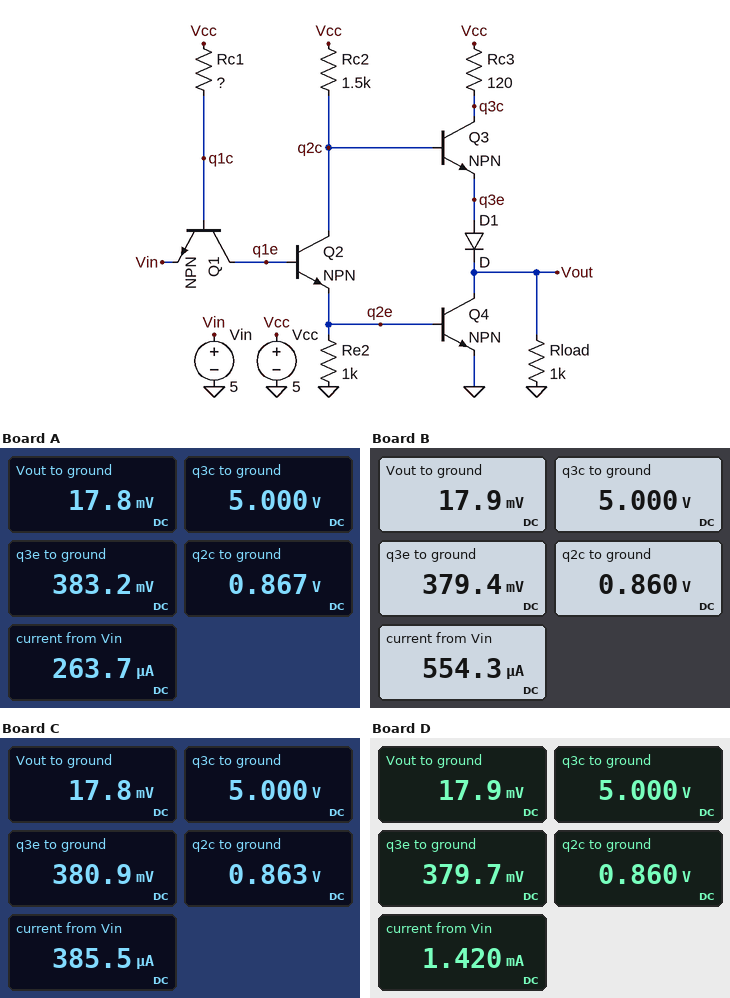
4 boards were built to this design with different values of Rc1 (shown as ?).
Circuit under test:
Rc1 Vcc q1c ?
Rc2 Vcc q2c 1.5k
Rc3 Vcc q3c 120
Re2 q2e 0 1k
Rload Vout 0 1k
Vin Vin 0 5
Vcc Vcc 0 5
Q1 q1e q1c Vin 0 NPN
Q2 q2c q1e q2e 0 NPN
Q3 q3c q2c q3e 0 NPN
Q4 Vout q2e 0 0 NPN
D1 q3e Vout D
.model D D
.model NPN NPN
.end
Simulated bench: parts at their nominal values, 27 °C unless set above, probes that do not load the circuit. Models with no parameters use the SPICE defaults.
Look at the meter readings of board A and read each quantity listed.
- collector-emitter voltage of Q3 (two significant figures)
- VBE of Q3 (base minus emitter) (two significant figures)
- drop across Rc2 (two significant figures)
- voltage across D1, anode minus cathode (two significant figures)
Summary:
4.6 V
480 mV
4.1 V
370 mV
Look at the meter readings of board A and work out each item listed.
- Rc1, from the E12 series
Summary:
10 kΩ
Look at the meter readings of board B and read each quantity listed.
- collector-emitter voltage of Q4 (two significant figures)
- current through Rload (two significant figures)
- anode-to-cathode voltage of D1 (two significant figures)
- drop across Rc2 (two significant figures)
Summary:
18 mV
18 µA
360 mV
4.1 V
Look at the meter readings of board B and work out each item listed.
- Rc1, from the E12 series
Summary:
4.7 kΩ
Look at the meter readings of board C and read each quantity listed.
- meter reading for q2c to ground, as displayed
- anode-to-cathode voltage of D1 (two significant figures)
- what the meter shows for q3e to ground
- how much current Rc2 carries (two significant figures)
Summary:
0.863 V
360 mV
380.9 mV
2.8 mA
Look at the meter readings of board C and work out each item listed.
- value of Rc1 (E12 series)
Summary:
6.8 kΩ
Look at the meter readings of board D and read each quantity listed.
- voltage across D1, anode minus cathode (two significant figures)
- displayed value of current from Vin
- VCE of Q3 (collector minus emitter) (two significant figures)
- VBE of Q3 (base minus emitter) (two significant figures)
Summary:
360 mV
1.420 mA
4.6 V
480 mV
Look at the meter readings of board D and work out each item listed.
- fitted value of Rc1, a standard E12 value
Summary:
1.8 kΩ
